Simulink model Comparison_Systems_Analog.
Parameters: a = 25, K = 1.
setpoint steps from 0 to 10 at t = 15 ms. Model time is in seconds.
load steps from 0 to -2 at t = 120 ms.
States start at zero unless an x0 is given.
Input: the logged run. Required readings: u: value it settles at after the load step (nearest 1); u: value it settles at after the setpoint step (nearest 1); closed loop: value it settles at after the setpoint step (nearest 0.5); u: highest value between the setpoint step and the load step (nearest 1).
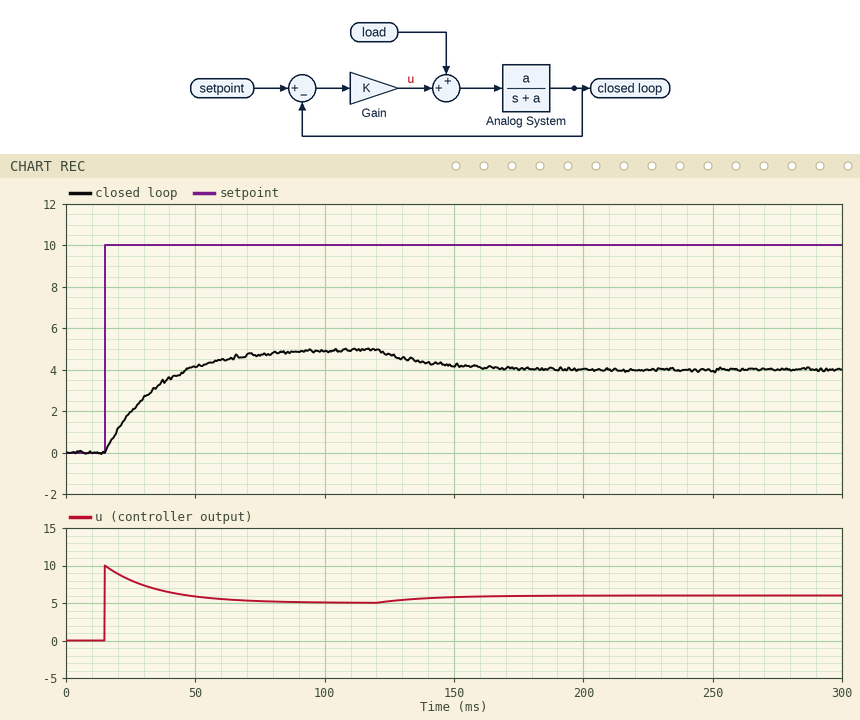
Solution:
6
5
5.0
10
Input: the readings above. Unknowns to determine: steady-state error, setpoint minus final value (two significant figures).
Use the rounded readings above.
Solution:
5.0
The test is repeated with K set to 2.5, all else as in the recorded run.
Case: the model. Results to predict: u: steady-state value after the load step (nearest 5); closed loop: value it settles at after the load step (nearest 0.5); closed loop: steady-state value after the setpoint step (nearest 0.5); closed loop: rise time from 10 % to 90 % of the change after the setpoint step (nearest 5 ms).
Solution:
10
6.5
7.0
25 ms
